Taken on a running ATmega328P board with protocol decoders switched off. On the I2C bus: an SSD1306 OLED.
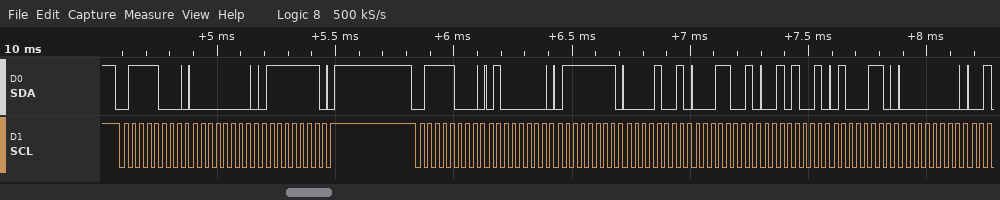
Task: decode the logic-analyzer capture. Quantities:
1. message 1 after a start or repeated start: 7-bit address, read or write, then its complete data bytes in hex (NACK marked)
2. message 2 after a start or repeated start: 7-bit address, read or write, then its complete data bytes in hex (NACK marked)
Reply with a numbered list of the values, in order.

1. 0x3C write: 00 7F
2. 0x3C write: 40 7F 09 19 29 46 00
